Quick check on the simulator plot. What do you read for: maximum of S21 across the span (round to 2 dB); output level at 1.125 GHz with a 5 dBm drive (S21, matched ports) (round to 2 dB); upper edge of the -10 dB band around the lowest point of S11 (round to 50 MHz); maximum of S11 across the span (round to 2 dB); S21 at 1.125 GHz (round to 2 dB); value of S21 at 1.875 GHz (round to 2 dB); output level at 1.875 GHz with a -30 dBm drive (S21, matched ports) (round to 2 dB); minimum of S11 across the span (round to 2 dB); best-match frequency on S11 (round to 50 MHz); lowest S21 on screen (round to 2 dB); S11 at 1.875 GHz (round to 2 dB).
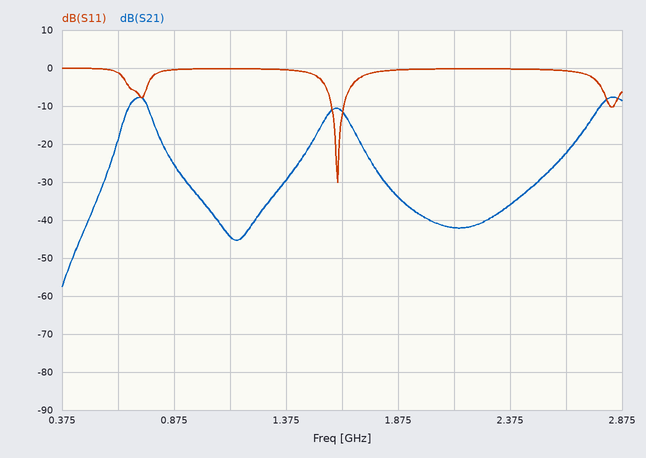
-8 dB
-40 dBm
1.65 GHz
0 dB
-44 dB
-34 dB
-64 dBm
-30 dB
1.60 GHz
-58 dB
0 dB
